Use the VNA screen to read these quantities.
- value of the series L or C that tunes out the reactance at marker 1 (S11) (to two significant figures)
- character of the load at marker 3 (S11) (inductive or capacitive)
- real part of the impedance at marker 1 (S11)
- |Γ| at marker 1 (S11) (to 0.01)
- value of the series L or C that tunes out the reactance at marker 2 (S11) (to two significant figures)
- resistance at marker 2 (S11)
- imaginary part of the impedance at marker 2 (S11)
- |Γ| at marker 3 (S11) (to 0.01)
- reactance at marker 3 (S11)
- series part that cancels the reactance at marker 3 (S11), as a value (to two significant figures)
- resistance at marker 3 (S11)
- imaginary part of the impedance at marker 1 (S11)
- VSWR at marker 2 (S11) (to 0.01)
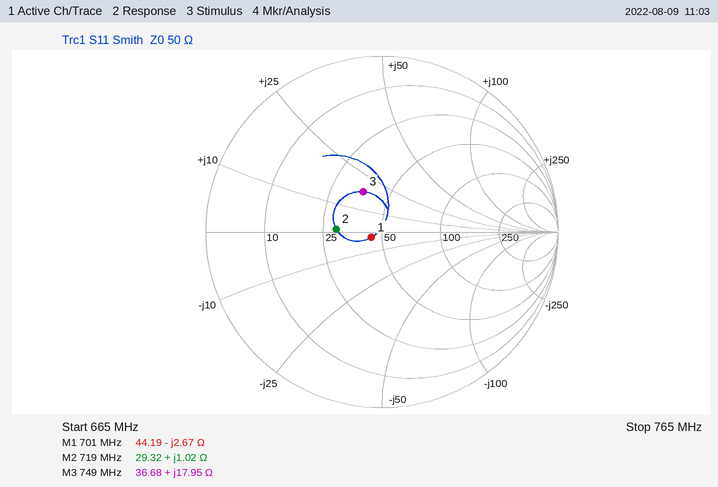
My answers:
610 pH
inductive
44.19 Ω
0.07
220 pF
29.32 Ω
+1.02 Ω
0.25
+17.95 Ω
12 pF
36.68 Ω
-2.67 Ω
1.71
